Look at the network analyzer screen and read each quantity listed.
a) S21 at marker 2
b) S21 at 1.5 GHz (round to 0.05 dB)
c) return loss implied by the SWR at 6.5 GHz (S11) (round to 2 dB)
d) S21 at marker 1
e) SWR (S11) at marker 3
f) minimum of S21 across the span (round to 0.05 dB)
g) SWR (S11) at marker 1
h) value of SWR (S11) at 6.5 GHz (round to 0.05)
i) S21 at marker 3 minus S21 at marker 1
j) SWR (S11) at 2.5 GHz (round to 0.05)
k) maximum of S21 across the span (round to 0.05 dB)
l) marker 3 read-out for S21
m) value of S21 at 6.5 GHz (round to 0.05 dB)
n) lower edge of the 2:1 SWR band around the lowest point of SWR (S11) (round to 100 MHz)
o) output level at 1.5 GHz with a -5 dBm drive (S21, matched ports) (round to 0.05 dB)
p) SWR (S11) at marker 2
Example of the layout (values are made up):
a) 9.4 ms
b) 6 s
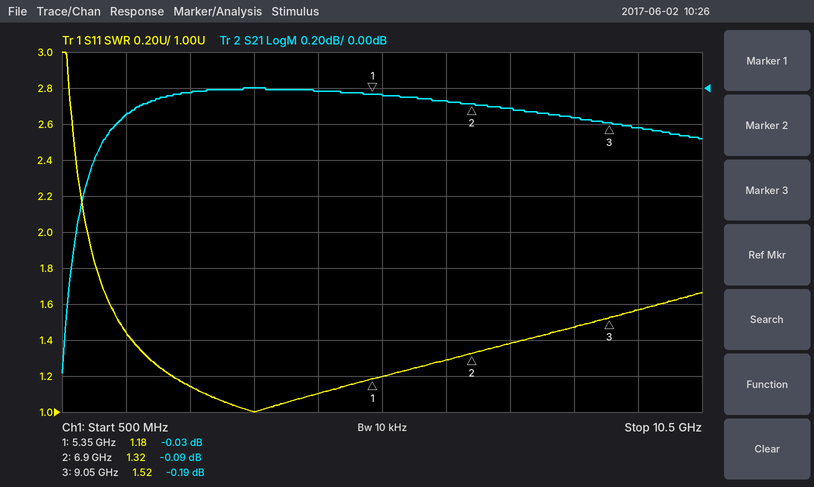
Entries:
a) -0.09 dB
b) -0.15 dB
c) 18 dB
d) -0.03 dB
e) 1.52
f) -1.60 dB
g) 1.18
h) 1.30
i) -0.16 dB
j) 1.15
k) 0.00 dB
l) -0.19 dB
m) -0.05 dB
n) 900 MHz
o) -5.15 dBm
p) 1.32
